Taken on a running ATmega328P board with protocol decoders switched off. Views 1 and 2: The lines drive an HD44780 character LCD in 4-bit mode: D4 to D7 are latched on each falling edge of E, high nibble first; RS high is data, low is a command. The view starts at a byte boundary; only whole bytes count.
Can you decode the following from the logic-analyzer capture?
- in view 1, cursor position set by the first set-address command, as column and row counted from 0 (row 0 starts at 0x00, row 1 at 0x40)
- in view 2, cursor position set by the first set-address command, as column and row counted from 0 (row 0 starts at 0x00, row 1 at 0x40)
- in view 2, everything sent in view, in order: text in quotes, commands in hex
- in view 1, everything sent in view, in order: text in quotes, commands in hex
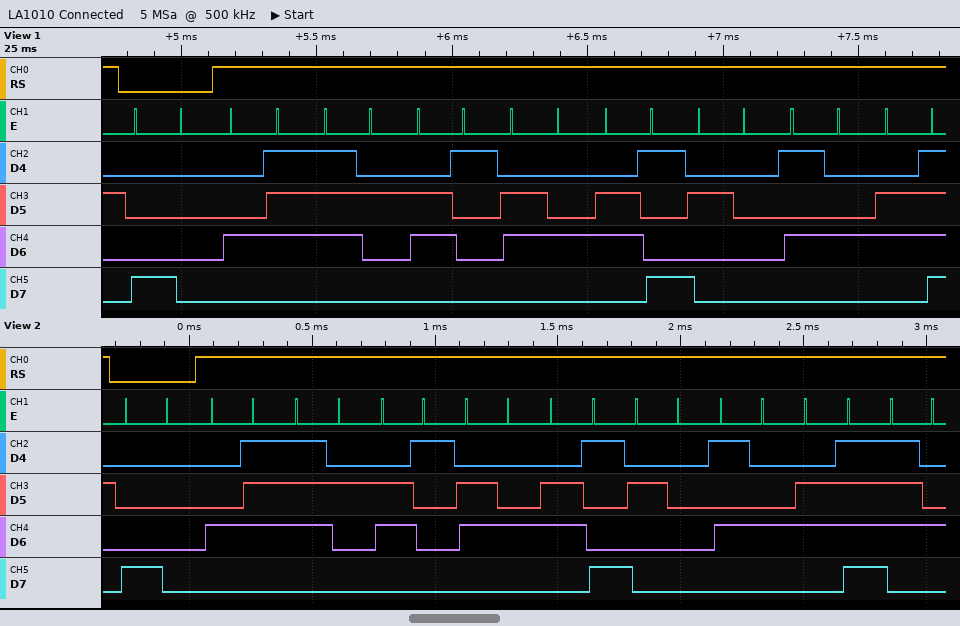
column 0, row 0
column 0, row 0
0x80 "Gradi Tot"
0x80 "Gradi To"
